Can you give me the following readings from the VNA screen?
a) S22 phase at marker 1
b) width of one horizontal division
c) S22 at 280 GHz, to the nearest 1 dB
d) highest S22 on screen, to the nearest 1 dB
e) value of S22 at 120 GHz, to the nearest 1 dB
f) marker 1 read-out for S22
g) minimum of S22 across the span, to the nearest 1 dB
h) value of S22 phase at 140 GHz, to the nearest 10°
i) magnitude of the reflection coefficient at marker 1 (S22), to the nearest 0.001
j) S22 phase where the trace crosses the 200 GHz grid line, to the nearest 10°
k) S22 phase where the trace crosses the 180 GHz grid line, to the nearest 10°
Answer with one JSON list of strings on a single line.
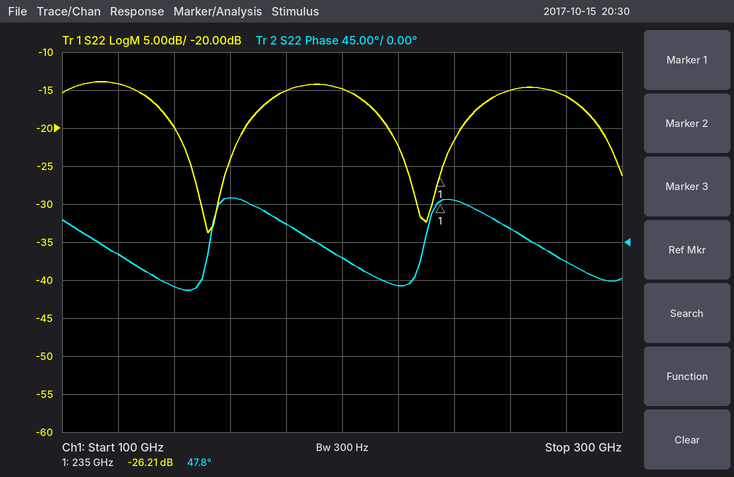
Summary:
["47.8°", "20 GHz", "-16 dB", "-14 dB", "-14 dB", "-26.21 dB", "-34 dB", "-50°", "0.049", "-20°", "20°"]
